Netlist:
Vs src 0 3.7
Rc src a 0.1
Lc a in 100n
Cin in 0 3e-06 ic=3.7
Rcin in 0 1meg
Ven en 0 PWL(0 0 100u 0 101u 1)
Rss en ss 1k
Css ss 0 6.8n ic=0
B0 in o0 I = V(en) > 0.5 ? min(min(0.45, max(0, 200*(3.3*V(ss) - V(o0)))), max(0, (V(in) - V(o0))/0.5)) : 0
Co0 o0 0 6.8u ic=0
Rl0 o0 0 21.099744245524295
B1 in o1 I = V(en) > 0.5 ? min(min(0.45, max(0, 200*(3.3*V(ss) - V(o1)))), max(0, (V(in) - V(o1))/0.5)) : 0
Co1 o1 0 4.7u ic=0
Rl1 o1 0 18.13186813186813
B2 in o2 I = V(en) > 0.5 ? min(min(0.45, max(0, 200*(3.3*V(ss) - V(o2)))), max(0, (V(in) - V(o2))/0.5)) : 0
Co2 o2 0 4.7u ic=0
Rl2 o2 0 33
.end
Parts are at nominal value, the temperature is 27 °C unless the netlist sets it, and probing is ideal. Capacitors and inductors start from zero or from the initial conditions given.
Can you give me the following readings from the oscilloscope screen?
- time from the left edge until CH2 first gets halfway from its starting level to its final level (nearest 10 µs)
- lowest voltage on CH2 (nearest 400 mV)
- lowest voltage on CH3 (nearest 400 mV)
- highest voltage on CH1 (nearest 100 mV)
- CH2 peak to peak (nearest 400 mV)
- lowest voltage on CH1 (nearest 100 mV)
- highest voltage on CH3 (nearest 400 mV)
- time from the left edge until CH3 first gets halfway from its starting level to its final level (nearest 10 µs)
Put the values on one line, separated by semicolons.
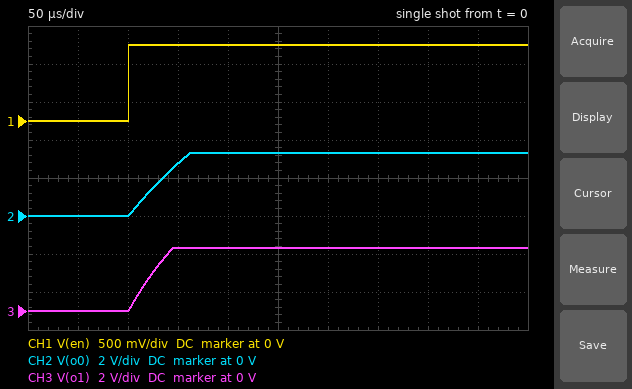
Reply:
130 µs; 0 V; 0 V; 1.0 V; 3.2 V; 0 V; 3.2 V; 120 µs
